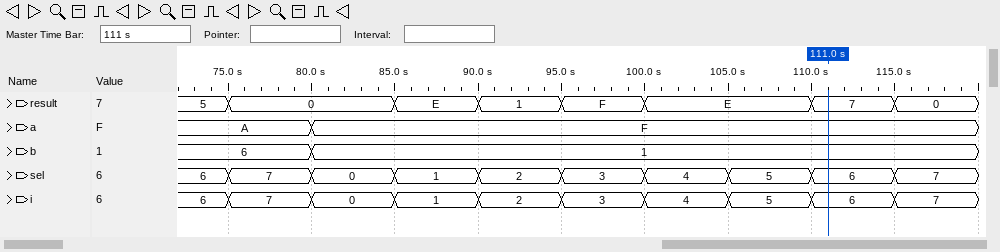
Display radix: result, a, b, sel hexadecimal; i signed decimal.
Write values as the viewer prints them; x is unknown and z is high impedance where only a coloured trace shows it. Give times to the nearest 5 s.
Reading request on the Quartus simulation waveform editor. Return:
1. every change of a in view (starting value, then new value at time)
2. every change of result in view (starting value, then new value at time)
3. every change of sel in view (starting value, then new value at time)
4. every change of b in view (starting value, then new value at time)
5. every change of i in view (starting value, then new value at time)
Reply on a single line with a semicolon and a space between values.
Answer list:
A, F at 80 s; 5, 0 at 75 s, E at 85 s, 1 at 90 s, F at 95 s, E at 100 s, 7 at 110 s, 0 at 115 s; 6, 7 at 75 s, 0 at 80 s, 1 at 85 s, 2 at 90 s, 3 at 95 s, 4 at 100 s, 5 at 105 s, 6 at 110 s, 7 at 115 s; 6, 1 at 80 s; 6, 7 at 75 s, 0 at 80 s, 1 at 85 s, 2 at 90 s, 3 at 95 s, 4 at 100 s, 5 at 105 s, 6 at 110 s, 7 at 115 s
